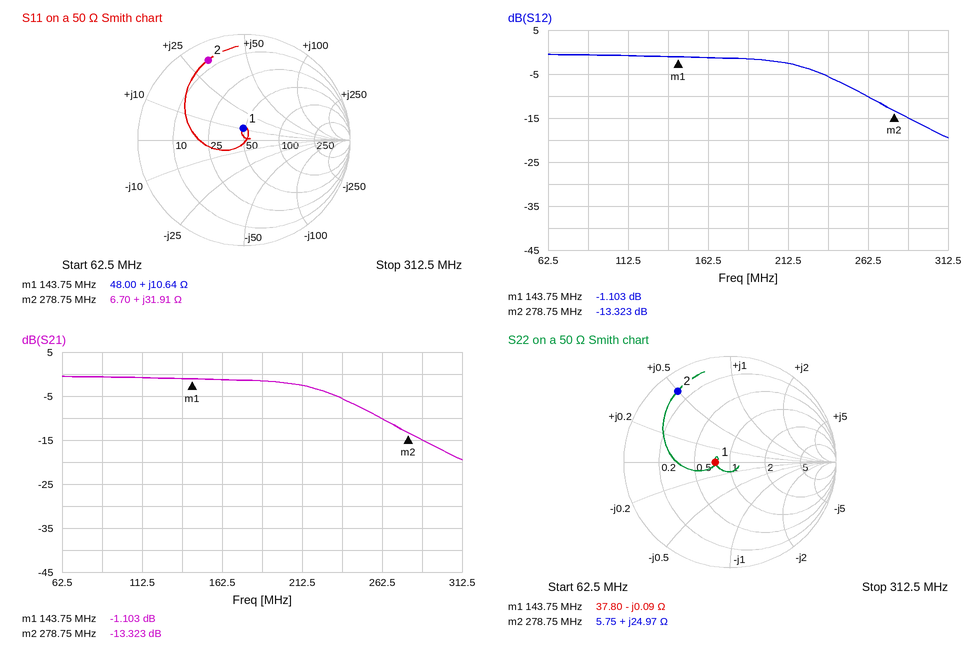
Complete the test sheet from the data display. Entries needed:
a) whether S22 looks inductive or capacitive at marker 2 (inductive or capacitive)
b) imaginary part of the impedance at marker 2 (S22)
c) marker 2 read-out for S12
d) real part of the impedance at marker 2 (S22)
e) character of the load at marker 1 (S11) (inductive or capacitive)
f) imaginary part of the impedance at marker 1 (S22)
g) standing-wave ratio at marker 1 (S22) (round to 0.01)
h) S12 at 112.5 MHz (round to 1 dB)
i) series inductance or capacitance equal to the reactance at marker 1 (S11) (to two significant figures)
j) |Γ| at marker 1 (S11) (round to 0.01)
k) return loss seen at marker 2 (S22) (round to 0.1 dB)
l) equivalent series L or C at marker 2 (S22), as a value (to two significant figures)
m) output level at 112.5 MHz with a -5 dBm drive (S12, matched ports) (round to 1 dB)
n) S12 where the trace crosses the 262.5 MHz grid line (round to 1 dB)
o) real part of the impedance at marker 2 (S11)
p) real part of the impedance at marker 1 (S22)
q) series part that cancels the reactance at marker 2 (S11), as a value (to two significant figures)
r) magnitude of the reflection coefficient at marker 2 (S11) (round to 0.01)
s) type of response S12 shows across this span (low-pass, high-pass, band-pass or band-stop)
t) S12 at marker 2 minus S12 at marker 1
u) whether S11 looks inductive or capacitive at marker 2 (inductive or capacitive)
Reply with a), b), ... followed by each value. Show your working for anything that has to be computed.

a) inductive
b) +24.97 Ω
c) -13.323 dB
d) 5.75 Ω
e) inductive
f) -0.09 Ω
g) 1.32
h) -1 dB
i) L = 10.64 Ω/(2π × 143.75 MHz) ≈ 12 nH
j) 0.11
k) 1.6 dB
l) L = 24.97 Ω/(2π × 278.75 MHz) ≈ 14 nH
m) -5 dBm + (-1 dB) = -6 dBm
n) -10 dB
o) 6.70 Ω
p) 37.80 Ω
q) C = 1/(2π × 278.75 MHz × 31.91 Ω) ≈ 18 pF
r) 0.83
s) low-pass
t) -13.323 − (-1.103) = -12.220 dB
u) inductive
